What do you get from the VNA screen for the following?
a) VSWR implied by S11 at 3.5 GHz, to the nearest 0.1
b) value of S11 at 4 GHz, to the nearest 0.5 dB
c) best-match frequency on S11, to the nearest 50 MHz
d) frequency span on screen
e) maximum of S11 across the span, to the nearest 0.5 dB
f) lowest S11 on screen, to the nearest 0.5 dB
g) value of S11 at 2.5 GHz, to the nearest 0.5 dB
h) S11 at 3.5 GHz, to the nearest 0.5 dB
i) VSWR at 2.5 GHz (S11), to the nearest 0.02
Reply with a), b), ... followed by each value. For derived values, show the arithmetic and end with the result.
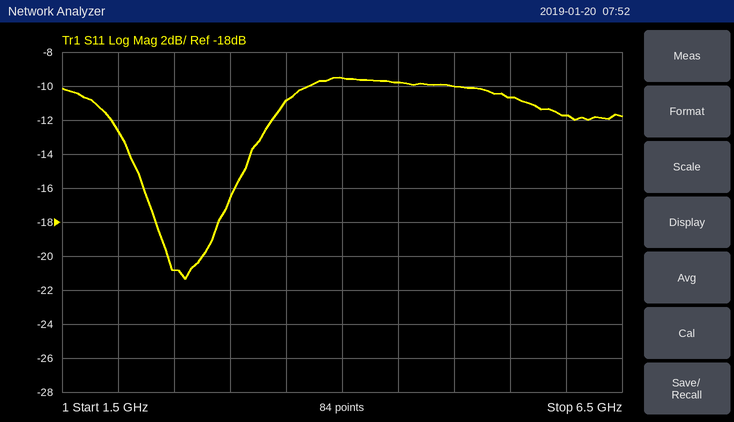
a) |Γ| = 10^(-11/20) = 0.2818; VSWR = (1 + 0.2818)/(1 − 0.2818) ≈ 1.8
b) -9.5 dB
c) 2.60 GHz
d) 5 GHz
e) -9.5 dB
f) -21.5 dB
g) -21.0 dB
h) -11.0 dB
i) |Γ| = 10^(-21/20) = 0.0891; VSWR = (1 + 0.0891)/(1 − 0.0891) ≈ 1.20
